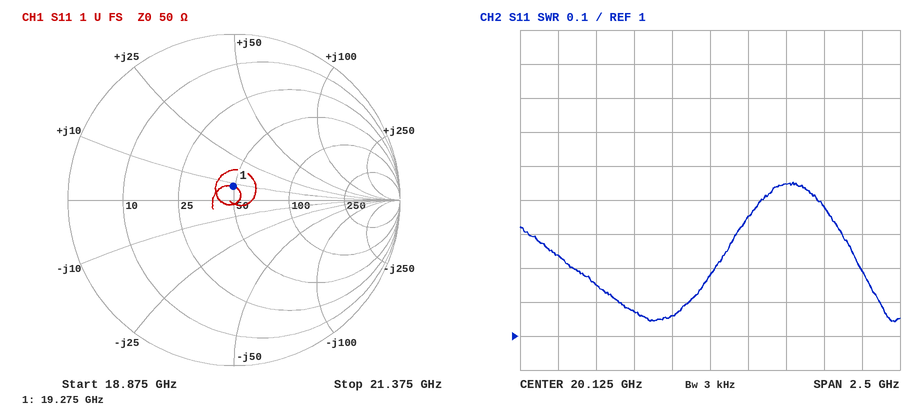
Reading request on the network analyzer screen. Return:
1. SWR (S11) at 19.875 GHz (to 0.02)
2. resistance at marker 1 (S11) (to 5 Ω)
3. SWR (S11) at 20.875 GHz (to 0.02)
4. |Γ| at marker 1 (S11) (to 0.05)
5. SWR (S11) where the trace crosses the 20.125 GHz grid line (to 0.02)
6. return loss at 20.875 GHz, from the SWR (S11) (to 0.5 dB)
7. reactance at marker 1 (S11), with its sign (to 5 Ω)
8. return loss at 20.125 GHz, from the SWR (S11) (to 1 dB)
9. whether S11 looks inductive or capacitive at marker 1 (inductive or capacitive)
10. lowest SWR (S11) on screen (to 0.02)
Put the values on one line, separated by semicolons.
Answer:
1.06; 50 Ω; 1.38; 0.10; 1.18; 16.0 dB; +10 Ω; 22 dB; inductive; 1.04
